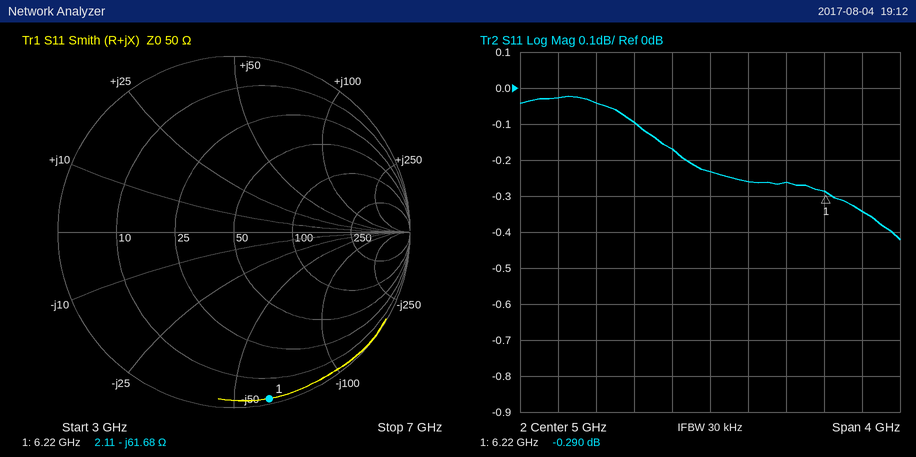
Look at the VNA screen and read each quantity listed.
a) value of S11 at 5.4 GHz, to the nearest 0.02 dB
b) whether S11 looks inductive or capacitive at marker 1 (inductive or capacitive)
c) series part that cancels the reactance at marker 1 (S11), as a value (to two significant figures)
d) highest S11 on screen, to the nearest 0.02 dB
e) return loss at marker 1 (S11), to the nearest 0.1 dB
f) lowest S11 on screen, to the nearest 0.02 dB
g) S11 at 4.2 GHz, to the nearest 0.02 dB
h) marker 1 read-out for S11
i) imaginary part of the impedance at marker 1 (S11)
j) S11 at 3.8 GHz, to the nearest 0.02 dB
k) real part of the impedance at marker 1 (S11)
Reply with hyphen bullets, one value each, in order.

- -0.26 dB
- capacitive
- 1.6 nH
- -0.02 dB
- 0.3 dB
- -0.42 dB
- -0.10 dB
- -0.290 dB
- -61.68 Ω
- -0.04 dB
- 2.11 Ω
